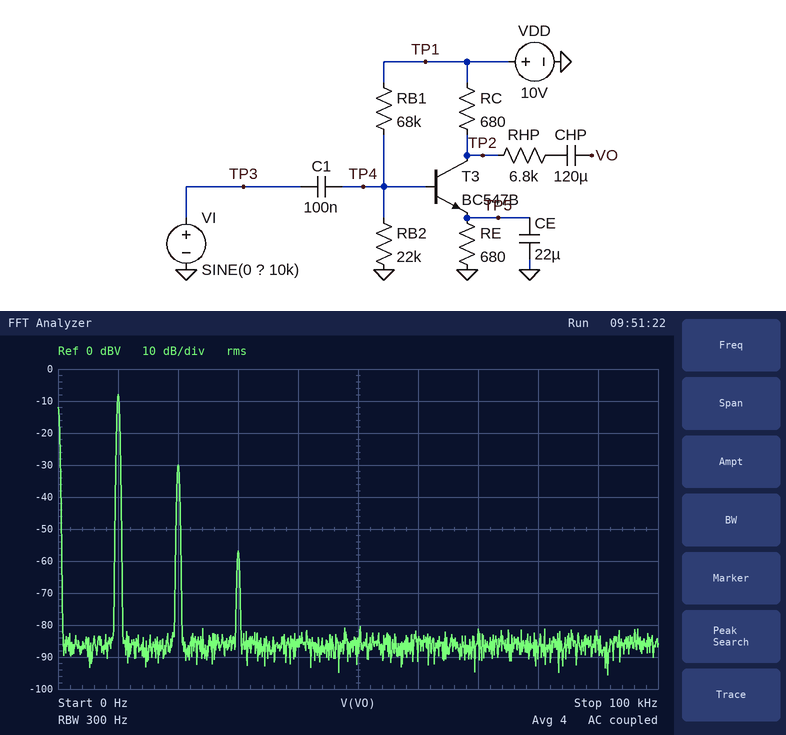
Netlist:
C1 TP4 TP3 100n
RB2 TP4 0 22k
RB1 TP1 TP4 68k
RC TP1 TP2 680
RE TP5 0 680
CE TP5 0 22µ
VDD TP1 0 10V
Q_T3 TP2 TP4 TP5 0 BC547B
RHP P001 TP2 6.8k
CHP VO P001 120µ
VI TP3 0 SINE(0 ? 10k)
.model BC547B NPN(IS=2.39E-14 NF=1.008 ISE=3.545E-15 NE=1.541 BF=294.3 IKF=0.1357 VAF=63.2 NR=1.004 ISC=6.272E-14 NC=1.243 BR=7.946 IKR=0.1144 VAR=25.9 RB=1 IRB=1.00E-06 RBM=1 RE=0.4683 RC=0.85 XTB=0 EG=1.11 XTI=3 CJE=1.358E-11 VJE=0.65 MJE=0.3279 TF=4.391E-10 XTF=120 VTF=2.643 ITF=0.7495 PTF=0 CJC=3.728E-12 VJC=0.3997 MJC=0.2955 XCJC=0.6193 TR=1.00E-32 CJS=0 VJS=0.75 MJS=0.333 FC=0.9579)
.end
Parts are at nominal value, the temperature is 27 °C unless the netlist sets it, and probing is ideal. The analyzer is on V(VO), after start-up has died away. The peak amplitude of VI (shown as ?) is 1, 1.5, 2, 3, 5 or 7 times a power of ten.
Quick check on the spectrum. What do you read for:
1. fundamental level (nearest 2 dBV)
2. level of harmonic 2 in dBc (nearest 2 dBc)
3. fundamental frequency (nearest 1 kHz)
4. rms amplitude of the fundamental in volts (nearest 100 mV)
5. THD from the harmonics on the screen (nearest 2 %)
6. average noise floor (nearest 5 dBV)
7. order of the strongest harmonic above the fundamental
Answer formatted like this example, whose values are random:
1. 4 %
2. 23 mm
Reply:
1. -8 dBV
2. -22 dBc
3. 10 kHz
4. 400 mV
5. 8 %
6. -85 dBV
7. 2
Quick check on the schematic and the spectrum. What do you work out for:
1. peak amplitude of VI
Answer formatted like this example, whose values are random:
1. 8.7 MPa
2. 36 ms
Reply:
1. 10 mV
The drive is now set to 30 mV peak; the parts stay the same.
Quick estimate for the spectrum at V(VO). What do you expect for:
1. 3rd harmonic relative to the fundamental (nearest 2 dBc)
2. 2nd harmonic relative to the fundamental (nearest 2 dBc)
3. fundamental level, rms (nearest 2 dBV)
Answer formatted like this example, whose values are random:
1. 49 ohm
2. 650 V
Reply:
1. -30 dBc
2. -12 dBc
3. 0 dBV
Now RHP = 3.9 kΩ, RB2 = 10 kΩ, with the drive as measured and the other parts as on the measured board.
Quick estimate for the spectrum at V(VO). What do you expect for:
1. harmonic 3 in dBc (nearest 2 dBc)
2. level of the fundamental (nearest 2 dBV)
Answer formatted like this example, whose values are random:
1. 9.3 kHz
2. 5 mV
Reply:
1. -46 dBc
2. -16 dBV
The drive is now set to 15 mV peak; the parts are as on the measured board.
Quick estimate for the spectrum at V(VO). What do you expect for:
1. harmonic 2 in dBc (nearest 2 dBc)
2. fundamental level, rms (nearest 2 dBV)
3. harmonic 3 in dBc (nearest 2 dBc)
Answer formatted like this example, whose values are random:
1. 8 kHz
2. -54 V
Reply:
1. -18 dBc
2. -4 dBV
3. -42 dBc
